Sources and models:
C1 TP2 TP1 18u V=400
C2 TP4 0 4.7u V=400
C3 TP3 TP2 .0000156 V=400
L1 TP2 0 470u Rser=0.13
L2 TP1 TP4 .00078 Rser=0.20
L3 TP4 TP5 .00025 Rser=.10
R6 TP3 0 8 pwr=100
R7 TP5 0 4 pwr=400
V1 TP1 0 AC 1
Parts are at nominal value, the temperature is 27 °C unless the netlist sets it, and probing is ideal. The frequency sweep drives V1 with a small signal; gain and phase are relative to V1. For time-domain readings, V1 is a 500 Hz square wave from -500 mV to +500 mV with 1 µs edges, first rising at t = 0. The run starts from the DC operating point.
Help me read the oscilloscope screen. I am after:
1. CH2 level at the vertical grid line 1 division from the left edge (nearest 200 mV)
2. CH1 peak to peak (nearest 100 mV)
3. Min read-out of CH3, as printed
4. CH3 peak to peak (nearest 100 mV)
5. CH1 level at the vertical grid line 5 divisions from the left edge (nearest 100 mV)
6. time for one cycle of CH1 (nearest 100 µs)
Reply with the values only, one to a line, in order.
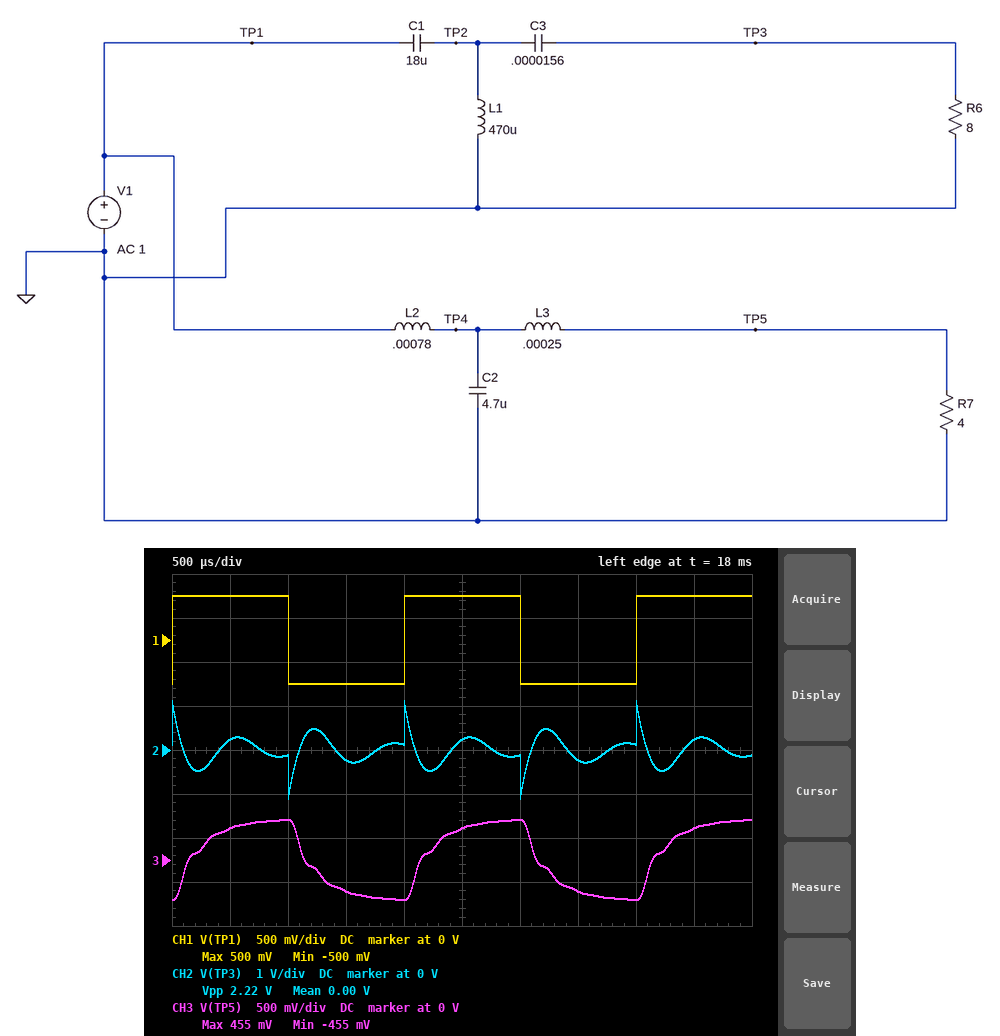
200 mV
1.0 V
-455 mV
900 mV
500 mV
2.0 ms
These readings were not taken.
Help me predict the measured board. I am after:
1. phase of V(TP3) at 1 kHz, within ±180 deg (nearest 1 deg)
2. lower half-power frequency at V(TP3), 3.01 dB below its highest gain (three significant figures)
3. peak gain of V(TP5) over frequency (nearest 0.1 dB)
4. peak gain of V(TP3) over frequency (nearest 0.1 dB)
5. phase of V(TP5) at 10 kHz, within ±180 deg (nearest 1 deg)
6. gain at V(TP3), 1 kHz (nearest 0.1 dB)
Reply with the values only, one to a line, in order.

-149 deg
1.29 kHz
-0.6 dB
4.3 dB
109 deg
-8.0 dB
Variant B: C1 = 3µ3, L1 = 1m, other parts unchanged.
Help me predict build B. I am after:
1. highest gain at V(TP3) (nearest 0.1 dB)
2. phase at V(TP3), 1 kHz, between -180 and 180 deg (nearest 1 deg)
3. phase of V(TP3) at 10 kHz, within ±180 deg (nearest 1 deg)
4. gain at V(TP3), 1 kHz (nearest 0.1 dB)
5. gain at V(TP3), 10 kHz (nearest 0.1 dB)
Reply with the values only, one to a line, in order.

0 dB
-161 deg
38 deg
-17.2 dB
-1.4 dB
